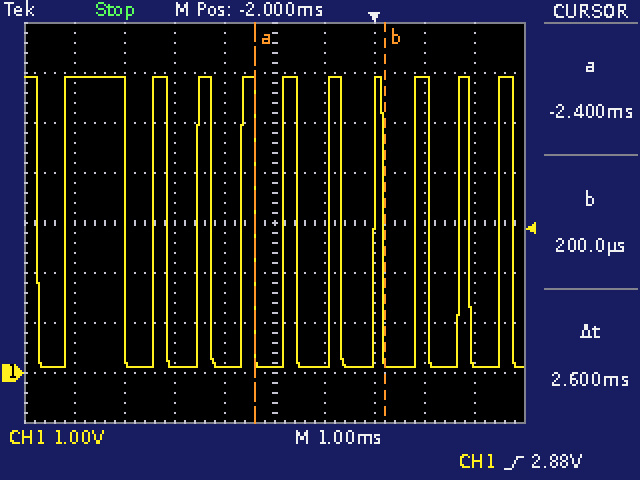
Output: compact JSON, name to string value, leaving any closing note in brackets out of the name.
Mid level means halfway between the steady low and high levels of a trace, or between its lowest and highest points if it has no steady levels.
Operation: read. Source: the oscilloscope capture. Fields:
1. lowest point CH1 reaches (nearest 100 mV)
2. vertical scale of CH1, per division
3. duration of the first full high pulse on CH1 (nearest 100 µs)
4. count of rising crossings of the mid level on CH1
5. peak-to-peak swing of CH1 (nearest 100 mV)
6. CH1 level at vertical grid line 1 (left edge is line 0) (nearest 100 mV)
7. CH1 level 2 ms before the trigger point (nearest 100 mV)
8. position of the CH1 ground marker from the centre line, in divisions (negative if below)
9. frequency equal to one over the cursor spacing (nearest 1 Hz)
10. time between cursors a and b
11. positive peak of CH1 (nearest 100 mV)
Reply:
{"lowest point CH1 reaches": "100 mV", "vertical scale of CH1, per division": "1 V", "duration of the first full high pulse on CH1": "1.2 ms", "count of rising crossings of the mid level on CH1": "10", "peak-to-peak swing of CH1": "5.8 V", "CH1 level at vertical grid line 1 (left edge is line 0)": "5.9 V", "CH1 level 2 ms before the trigger point": "100 mV", "position of the CH1 ground marker from the centre line, in divisions": "-3.0 div", "frequency equal to one over the cursor spacing": "385 Hz", "time between cursors a and b": "2.6 ms", "positive peak of CH1": "5.9 V"}
